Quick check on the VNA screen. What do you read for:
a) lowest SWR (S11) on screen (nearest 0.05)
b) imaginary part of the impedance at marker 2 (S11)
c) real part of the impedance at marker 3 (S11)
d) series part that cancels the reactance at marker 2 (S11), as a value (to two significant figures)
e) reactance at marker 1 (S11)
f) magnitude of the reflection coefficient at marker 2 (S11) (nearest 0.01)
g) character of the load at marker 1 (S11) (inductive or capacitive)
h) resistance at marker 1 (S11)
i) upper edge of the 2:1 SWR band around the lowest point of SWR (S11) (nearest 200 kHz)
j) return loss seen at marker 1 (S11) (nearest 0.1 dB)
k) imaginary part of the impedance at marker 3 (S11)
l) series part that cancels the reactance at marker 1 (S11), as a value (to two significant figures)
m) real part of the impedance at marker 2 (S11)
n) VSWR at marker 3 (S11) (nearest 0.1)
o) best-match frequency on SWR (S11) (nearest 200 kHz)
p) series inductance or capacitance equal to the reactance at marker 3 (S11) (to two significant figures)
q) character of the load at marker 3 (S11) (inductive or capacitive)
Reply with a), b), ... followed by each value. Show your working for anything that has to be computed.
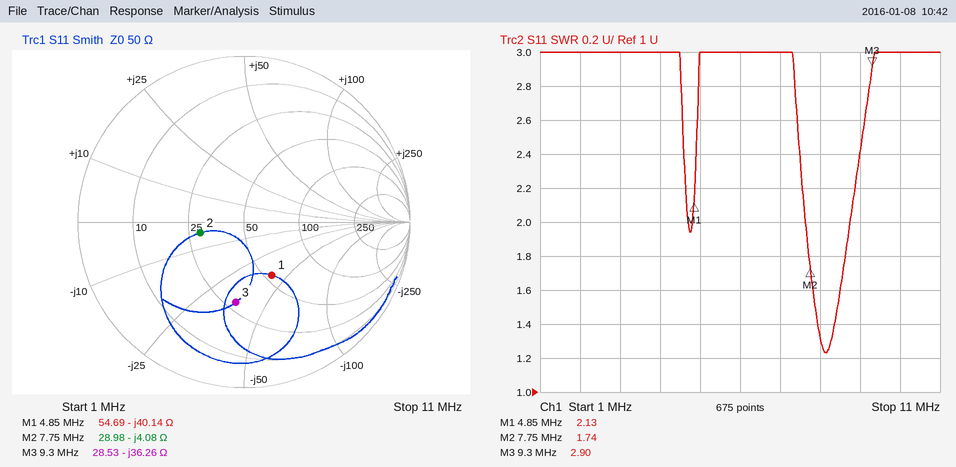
a) 1.25
b) -4.08 Ω
c) 28.53 Ω
d) L = 4.08 Ω/(2π × 7.75 MHz) ≈ 84 nH
e) -40.14 Ω
f) 0.27
g) capacitive
h) 54.69 Ω
i) 8.8 MHz
j) 8.9 dB
k) -36.26 Ω
l) L = 40.14 Ω/(2π × 4.85 MHz) ≈ 1.3 µH
m) 28.98 Ω
n) 2.9
o) 8.2 MHz
p) C = 1/(2π × 9.3 MHz × 36.26 Ω) ≈ 472 pF, so 470 pF to two significant figures
q) capacitive
